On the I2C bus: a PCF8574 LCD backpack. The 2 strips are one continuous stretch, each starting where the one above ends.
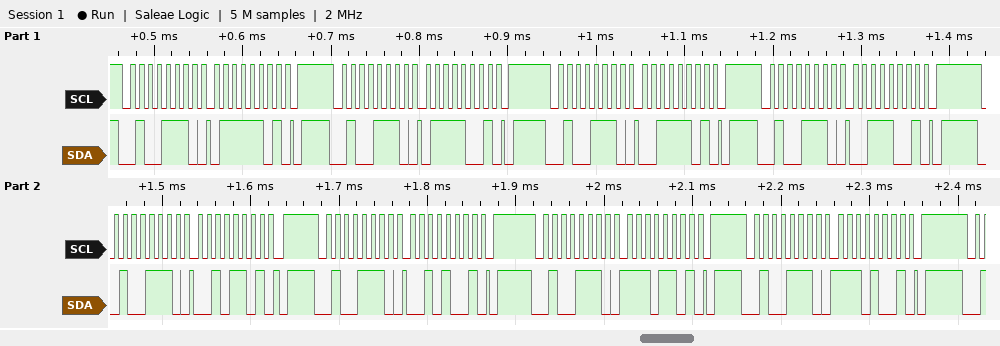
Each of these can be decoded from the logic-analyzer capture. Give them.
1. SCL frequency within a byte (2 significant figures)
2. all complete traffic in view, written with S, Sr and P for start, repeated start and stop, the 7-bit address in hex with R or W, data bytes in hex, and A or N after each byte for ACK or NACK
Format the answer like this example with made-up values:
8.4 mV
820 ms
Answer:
100 kHz
S 27W A 7D A P S 27W A 79 A P S 27W A 3D A P S 27W A 39 A P S 27W A 2D A P S 27W A 29 A P S 27W A ED A P S 27W A E9 A P
